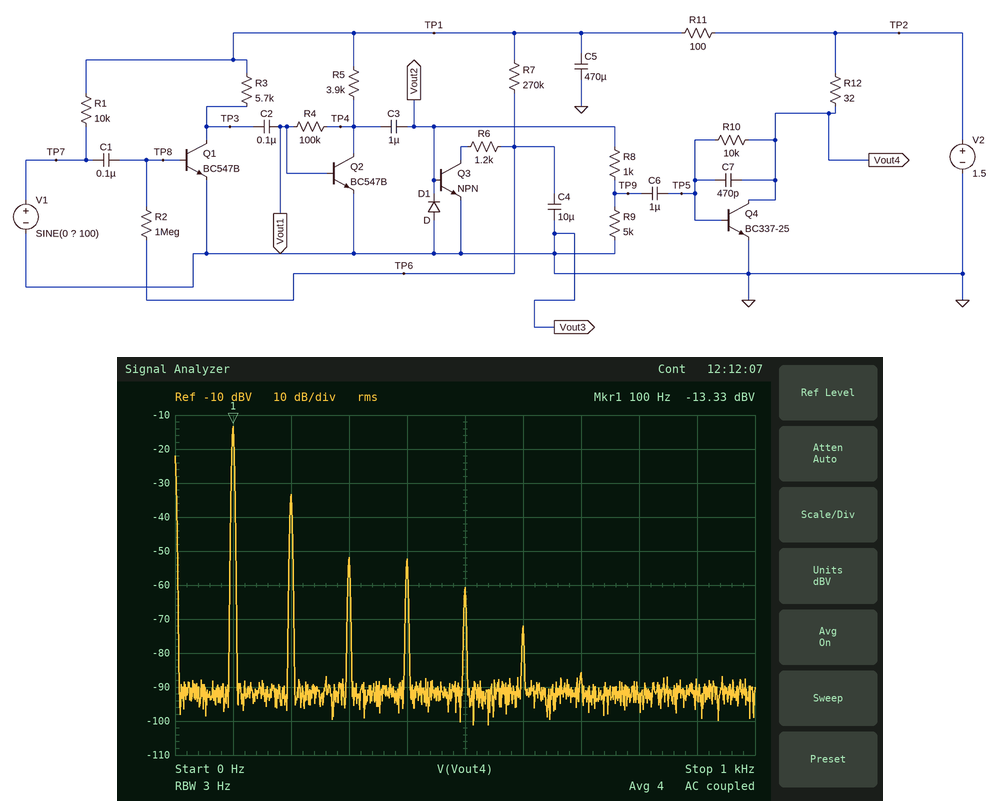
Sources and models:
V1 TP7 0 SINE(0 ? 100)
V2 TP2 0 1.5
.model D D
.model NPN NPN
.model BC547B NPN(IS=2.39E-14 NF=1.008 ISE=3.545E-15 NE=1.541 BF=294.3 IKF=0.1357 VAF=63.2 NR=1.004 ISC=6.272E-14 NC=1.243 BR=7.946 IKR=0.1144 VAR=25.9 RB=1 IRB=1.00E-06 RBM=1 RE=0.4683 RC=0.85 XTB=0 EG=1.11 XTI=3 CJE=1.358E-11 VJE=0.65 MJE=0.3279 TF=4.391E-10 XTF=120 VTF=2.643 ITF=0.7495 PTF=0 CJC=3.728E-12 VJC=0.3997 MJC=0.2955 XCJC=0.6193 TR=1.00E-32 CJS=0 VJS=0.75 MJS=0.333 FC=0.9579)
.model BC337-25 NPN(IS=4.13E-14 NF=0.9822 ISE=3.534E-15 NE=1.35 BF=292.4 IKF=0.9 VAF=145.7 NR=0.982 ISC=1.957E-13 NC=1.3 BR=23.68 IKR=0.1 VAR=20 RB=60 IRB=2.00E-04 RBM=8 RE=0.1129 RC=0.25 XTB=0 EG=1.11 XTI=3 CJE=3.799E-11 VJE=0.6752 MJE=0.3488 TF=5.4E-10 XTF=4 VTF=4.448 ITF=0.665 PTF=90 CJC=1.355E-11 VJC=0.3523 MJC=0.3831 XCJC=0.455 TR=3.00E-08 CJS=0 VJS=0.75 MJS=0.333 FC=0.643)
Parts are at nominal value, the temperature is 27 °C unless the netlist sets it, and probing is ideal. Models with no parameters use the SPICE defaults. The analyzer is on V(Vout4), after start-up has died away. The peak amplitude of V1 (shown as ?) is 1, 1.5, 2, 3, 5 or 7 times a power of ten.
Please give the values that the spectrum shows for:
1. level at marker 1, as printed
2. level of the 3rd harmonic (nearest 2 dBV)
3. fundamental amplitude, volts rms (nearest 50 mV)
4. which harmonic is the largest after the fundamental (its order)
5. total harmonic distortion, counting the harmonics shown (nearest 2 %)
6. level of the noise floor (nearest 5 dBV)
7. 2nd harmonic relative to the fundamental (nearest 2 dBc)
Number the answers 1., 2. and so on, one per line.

1. -13.33 dBV
2. -52 dBV
3. 200 mV
4. 2
5. 10 %
6. -90 dBV
7. -20 dBc
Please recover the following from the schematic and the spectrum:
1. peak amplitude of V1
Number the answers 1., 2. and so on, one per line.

1. 1.5 mV
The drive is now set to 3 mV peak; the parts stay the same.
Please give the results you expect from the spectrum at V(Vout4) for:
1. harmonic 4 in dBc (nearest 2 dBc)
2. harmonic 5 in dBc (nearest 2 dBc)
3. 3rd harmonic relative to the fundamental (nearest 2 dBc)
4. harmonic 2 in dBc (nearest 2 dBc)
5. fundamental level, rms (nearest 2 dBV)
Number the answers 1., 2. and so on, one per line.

1. -22 dBc
2. -40 dBc
3. -18 dBc
4. -16 dBc
5. -10 dBV
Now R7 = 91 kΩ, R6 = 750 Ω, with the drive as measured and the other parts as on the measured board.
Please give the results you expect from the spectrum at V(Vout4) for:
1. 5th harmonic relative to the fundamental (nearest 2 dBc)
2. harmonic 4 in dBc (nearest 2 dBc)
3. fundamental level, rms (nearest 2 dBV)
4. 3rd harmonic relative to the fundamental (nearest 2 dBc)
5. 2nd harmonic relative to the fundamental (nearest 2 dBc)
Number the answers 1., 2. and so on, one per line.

1. -44 dBc
2. -38 dBc
3. -14 dBV
4. -30 dBc
5. -22 dBc
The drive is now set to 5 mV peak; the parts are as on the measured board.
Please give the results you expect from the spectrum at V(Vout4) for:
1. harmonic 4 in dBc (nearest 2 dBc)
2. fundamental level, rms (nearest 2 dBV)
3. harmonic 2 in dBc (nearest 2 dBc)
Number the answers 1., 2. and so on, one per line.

1. -18 dBc
2. -10 dBV
3. -10 dBc
